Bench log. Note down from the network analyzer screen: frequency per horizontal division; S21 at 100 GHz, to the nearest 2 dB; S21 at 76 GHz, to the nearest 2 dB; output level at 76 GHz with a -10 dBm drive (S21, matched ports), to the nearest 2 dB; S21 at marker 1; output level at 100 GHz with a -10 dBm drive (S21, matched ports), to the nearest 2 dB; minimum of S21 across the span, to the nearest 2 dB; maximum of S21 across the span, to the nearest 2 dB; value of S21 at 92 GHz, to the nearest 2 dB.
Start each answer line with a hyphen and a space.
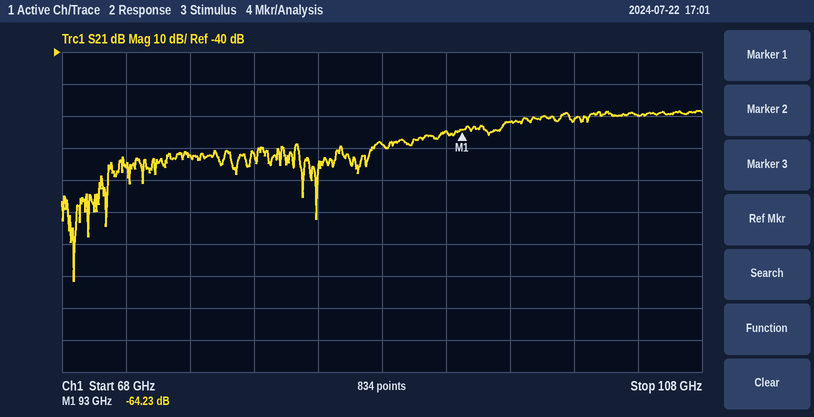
- 4 GHz
- -62 dB
- -72 dB
- -82 dBm
- -64.23 dB
- -72 dBm
- -112 dB
- -58 dB
- -64 dB
